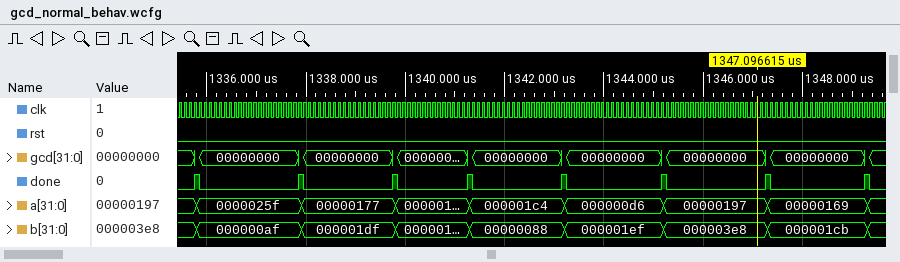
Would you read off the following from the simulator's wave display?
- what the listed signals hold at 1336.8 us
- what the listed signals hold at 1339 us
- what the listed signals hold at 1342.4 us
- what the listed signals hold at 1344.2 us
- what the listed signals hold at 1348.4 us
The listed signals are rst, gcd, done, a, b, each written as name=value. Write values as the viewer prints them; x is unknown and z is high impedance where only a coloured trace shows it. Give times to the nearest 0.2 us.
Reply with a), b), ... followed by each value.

a) rst=0, gcd=00000000, done=0, a=0000025f, b=000000af
b) rst=0, gcd=00000000, done=0, a=00000177, b=000001df
c) rst=0, gcd=00000000, done=0, a=000001c4, b=00000088
d) rst=0, gcd=00000000, done=0, a=000000d6, b=000001ef
e) rst=0, gcd=00000000, done=0, a=00000169, b=000001cb
